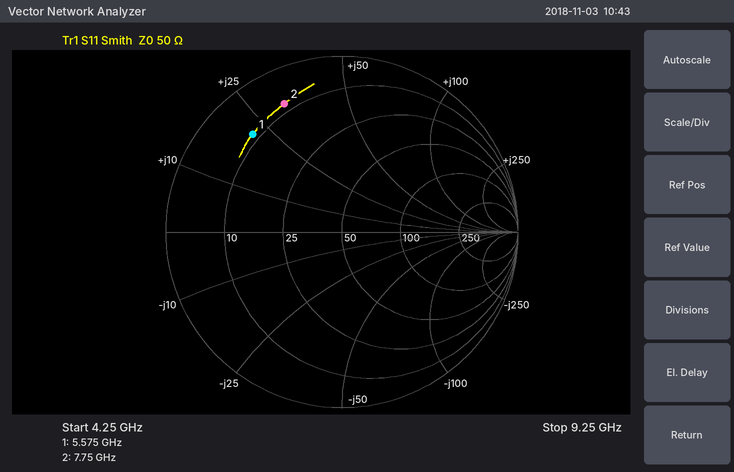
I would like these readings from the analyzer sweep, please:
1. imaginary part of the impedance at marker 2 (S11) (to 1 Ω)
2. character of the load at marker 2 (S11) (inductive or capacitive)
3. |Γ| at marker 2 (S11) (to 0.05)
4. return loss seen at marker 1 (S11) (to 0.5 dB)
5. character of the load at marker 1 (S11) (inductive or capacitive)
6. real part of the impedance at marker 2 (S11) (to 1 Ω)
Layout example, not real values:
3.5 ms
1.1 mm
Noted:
+32 Ω
inductive
0.80
2.5 dB
inductive
8 Ω
